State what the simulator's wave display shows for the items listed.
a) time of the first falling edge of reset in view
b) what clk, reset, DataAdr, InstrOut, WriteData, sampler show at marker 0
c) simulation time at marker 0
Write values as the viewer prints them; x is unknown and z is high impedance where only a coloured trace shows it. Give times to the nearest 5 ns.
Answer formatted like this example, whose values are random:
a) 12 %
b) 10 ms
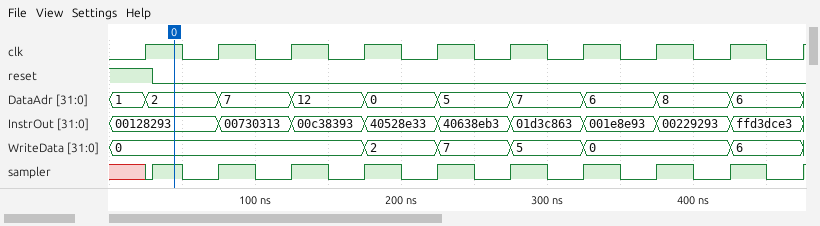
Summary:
a) 30 ns
b) clk=1, reset=0, DataAdr=2, InstrOut=00128293, WriteData=0, sampler=1
c) 45 ns
